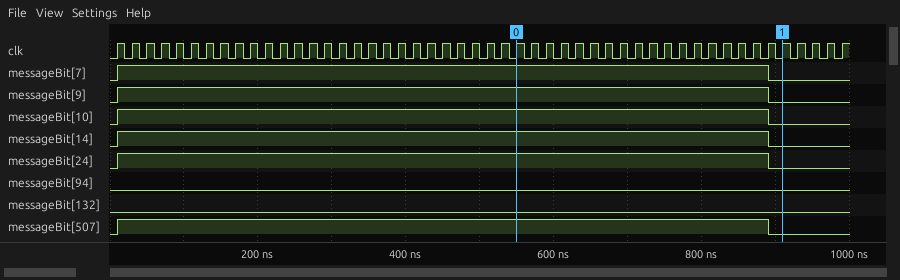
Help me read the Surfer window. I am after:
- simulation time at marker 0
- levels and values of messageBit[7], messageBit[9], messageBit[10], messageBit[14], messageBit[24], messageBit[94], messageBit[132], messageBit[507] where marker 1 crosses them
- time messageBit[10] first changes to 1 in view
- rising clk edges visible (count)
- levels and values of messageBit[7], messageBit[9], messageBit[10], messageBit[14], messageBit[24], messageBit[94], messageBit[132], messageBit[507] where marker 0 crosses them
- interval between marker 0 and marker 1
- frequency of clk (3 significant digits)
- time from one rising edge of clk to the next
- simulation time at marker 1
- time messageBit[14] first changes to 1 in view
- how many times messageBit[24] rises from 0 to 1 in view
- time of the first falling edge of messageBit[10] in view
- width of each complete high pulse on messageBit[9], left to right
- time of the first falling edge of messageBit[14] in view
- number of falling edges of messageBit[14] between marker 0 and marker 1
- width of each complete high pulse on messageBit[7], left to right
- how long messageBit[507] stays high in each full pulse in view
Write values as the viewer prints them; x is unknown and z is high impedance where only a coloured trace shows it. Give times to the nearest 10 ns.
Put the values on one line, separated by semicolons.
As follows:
550 ns; messageBit[7]=0, messageBit[9]=0, messageBit[10]=0, messageBit[14]=0, messageBit[24]=0, messageBit[94]=0, messageBit[132]=0, messageBit[507]=0; 10 ns; 50; messageBit[7]=1, messageBit[9]=1, messageBit[10]=1, messageBit[14]=1, messageBit[24]=1, messageBit[94]=0, messageBit[132]=0, messageBit[507]=1; 360 ns; 50.0 MHz; 20 ns; 910 ns; 10 ns; 1; 890 ns; 880 ns; 890 ns; 1; 880 ns; 880 ns
